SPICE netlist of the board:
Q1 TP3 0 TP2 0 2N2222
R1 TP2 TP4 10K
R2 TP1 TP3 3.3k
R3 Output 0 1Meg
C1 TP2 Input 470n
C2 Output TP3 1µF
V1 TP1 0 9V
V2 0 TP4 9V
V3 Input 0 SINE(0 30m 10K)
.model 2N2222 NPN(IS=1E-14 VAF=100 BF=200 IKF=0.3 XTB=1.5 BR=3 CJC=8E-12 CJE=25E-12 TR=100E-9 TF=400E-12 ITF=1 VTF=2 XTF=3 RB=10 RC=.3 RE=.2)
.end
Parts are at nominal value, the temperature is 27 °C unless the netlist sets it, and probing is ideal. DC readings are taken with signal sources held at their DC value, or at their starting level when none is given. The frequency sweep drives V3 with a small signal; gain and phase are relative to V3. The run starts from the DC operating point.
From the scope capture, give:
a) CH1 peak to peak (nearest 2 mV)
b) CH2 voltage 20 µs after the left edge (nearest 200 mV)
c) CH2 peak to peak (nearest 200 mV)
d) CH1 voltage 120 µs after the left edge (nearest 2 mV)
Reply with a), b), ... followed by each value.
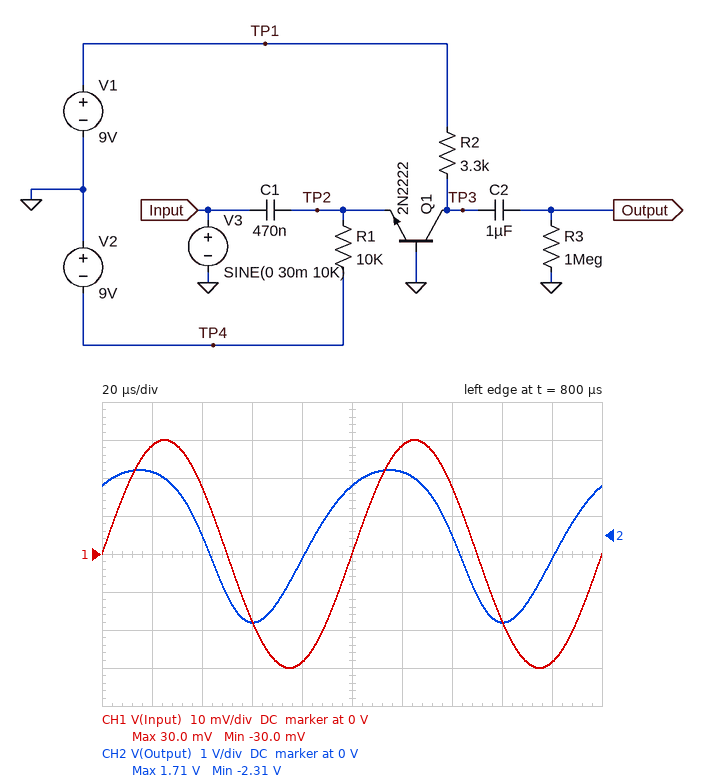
a) 60 mV
b) 1.6 V
c) 4.0 V
d) 28 mV
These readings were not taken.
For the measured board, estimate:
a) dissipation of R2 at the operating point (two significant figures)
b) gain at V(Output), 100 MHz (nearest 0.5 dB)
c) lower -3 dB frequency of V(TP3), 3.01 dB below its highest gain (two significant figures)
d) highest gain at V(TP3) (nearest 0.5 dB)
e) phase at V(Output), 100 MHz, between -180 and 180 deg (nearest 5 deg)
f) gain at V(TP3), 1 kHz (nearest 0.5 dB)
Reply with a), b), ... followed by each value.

a) 2.3 mW
b) 19.5 dB
c) 11 kHz
d) 40.0 dB
e) -95 deg
f) 19.5 dB
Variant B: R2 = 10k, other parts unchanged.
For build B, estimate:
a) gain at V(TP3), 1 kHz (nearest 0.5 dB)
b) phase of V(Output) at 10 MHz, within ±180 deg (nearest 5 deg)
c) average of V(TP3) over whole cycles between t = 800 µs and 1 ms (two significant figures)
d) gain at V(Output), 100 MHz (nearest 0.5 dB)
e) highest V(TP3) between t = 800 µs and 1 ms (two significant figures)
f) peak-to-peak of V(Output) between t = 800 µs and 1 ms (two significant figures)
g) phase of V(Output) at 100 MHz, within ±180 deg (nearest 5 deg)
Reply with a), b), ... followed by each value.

a) 29.0 dB
b) -80 deg
c) 1.5 V
d) 15.0 dB
e) 5.3 V
f) 6.0 V
g) -100 deg
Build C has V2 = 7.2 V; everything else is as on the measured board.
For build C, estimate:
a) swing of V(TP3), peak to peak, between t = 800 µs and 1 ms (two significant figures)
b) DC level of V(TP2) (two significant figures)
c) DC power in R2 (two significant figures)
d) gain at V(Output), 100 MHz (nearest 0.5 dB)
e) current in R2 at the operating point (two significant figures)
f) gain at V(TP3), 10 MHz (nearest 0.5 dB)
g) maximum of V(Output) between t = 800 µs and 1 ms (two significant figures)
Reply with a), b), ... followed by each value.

a) 3.5 V
b) -640 mV
c) 1.4 mW
d) 18.0 dB
e) 650 µA
f) 35.5 dB
g) 1.4 V
